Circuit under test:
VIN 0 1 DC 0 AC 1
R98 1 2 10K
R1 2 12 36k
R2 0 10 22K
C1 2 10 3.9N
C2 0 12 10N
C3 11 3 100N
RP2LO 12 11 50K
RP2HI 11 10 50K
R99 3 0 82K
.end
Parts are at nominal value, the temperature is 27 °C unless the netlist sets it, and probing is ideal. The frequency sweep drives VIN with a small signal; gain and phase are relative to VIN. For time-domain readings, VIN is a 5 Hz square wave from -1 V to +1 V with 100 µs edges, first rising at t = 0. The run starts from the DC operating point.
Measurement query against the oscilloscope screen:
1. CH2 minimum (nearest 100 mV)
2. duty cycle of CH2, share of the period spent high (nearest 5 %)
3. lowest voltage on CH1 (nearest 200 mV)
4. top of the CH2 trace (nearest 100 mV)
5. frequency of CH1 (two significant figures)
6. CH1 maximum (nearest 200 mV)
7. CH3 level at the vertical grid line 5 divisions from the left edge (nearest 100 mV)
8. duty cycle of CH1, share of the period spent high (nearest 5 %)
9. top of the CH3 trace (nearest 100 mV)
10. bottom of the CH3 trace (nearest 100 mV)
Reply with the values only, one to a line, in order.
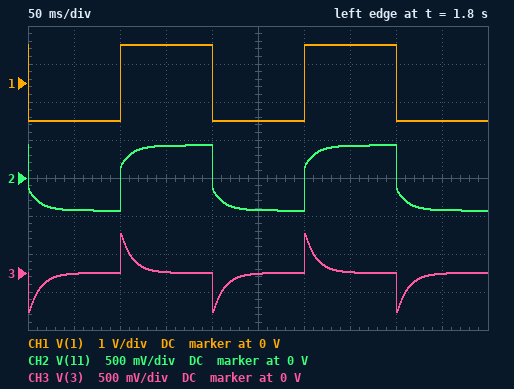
-400 mV
50 %
-1.0 V
400 mV
5.0 Hz
1.0 V
0 V
50 %
500 mV
-500 mV
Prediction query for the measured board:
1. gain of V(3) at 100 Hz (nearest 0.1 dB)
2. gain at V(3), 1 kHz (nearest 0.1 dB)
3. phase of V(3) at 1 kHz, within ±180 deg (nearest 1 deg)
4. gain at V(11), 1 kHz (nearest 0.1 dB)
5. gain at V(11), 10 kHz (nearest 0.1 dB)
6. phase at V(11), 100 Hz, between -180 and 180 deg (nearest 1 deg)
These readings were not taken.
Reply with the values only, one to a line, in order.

-11.2 dB
-18.7 dB
168 deg
-18.7 dB
-13.9 dB
168 deg
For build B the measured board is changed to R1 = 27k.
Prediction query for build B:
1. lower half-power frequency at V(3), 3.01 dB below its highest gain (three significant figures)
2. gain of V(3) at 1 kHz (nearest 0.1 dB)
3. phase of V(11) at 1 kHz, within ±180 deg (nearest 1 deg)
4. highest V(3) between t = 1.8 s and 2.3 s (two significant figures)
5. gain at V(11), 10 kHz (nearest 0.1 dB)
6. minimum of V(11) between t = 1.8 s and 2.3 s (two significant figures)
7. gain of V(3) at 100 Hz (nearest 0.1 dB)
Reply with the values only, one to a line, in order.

12.5 Hz
-17.2 dB
159 deg
560 mV
-14.3 dB
-450 mV
-10.5 dB
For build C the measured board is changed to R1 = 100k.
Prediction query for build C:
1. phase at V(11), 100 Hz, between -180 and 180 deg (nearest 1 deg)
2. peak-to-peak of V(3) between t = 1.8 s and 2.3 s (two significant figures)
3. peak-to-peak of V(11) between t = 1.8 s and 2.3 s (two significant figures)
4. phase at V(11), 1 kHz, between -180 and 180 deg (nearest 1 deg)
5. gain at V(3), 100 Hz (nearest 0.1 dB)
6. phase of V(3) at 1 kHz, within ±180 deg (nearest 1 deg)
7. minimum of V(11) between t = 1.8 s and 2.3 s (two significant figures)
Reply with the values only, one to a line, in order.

164 deg
670 mV
620 mV
-153 deg
-14.9 dB
-152 deg
-310 mV
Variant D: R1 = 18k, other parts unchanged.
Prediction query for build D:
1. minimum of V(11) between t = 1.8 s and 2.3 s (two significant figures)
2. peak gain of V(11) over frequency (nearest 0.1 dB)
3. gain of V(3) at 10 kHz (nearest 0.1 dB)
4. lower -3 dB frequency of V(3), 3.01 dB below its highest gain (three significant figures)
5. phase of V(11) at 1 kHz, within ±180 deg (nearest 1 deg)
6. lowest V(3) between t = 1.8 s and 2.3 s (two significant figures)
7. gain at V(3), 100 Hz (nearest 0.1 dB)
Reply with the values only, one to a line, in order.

-480 mV
-6.4 dB
-15.1 dB
12.8 Hz
153 deg
-610 mV
-9.8 dB
